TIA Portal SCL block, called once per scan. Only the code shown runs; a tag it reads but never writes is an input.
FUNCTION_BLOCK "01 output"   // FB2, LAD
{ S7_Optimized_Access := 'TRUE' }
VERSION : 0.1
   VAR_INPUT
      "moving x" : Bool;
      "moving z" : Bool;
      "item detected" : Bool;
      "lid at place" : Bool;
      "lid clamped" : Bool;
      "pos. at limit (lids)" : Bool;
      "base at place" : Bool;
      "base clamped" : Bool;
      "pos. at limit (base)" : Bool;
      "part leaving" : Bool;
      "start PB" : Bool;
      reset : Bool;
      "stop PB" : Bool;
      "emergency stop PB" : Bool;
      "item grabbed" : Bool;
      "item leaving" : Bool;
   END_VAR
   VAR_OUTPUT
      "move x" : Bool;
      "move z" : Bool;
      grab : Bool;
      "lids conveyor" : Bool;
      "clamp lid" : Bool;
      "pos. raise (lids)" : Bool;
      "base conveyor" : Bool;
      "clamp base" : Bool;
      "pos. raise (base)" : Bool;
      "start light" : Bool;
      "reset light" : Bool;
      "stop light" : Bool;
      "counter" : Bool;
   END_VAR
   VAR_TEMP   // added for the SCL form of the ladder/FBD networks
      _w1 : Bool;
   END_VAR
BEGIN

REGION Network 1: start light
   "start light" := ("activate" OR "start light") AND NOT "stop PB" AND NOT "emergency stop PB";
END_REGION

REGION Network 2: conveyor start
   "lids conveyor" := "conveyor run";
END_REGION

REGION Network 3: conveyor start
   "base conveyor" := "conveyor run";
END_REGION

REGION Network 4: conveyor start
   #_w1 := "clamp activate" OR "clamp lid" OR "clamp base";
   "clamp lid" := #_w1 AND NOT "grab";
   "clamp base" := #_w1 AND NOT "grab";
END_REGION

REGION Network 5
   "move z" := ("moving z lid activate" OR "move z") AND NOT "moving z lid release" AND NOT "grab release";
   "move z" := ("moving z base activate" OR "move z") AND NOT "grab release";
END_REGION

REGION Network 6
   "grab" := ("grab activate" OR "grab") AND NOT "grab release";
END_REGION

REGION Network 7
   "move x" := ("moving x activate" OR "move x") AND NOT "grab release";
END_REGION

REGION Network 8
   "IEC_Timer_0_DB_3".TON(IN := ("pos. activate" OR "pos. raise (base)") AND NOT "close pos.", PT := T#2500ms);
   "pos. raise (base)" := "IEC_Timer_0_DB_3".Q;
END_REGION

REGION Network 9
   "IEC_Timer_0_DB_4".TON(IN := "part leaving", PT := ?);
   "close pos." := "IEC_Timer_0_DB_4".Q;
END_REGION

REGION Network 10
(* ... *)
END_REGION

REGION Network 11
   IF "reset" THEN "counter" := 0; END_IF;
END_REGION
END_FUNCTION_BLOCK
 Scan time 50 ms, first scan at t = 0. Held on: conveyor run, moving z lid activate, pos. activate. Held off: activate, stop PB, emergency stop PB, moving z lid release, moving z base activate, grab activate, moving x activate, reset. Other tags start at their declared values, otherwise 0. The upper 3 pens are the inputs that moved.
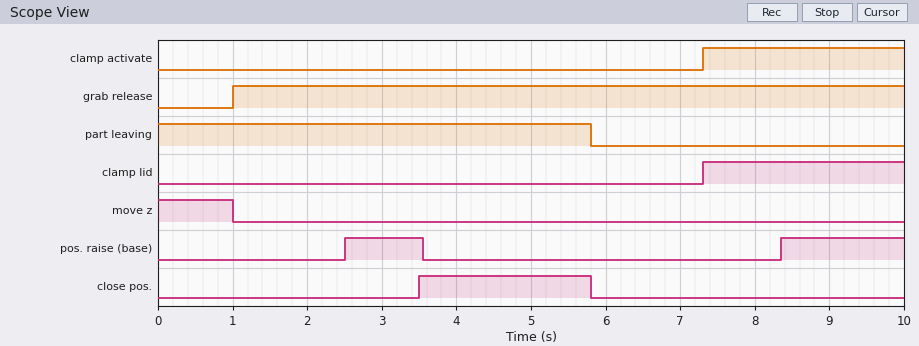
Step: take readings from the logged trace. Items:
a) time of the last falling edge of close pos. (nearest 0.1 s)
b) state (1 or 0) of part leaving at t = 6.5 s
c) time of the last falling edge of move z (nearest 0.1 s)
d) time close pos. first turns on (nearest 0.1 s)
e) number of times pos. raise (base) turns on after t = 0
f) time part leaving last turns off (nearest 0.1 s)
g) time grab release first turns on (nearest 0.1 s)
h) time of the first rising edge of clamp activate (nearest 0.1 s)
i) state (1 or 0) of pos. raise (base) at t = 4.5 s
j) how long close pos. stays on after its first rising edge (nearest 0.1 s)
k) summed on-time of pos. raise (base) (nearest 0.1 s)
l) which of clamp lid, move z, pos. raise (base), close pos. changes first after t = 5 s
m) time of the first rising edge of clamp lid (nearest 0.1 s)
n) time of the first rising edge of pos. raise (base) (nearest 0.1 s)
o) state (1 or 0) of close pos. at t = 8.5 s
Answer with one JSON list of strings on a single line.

["5.8 s", "0", "1.0 s", "3.5 s", "2", "5.8 s", "1.0 s", "7.3 s", "0", "2.3 s", "2.7 s", "close pos.", "7.3 s", "2.5 s", "0"]
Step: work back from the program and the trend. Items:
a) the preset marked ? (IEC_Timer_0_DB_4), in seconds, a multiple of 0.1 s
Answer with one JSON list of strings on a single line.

["3.5 s"]
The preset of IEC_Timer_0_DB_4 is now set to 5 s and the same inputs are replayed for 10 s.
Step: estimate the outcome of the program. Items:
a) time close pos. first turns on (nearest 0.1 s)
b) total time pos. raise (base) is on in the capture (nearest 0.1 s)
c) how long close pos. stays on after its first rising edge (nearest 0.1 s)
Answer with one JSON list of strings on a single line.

["5.0 s", "4.2 s", "0.8 s"]
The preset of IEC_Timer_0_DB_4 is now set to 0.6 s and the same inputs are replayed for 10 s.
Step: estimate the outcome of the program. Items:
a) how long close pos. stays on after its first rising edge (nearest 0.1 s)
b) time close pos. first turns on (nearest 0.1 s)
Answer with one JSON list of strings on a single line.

["5.2 s", "0.6 s"]
